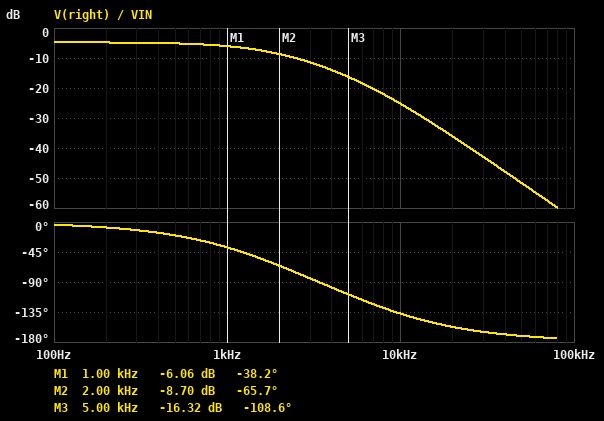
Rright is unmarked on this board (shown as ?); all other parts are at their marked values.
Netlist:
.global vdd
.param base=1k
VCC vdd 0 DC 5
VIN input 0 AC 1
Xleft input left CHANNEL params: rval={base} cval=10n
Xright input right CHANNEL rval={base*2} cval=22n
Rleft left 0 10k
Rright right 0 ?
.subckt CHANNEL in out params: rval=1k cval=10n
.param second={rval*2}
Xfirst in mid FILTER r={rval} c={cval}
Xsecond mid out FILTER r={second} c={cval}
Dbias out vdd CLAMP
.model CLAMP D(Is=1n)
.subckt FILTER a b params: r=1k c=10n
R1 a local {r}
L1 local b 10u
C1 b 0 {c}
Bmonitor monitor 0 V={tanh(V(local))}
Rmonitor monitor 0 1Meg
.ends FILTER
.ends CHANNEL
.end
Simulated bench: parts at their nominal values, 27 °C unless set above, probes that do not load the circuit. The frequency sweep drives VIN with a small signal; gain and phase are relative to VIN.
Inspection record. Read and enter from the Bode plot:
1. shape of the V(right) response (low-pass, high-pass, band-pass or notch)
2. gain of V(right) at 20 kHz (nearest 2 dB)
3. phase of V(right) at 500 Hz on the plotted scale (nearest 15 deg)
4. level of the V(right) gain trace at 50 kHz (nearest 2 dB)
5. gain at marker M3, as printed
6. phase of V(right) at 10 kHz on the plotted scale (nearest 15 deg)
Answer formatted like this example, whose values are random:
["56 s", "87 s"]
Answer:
["low-pass", "-36 dB", "-15 deg", "-52 dB", "-16.32 dB", "-135 deg"]
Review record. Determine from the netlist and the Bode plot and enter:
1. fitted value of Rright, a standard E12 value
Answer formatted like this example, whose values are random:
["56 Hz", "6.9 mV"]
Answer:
["8.2 kΩ"]
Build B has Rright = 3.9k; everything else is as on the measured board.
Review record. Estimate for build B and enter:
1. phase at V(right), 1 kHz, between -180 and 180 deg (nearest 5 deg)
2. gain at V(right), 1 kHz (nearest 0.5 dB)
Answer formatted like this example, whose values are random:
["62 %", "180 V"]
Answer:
["-30 deg", "-9.0 dB"]
